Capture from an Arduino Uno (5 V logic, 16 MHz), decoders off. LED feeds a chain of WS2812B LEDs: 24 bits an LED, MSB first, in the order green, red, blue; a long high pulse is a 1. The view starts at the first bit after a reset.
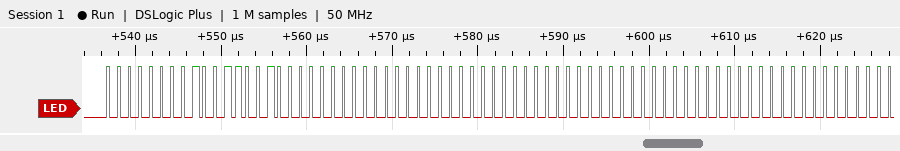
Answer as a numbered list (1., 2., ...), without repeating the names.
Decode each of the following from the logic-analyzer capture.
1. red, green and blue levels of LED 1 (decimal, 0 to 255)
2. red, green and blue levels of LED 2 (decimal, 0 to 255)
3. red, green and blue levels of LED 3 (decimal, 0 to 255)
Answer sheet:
1. 153, 0, 0
2. 0, 0, 0
3. 0, 0, 0
